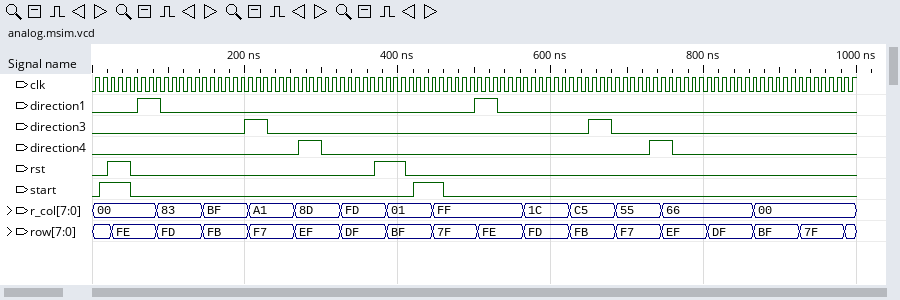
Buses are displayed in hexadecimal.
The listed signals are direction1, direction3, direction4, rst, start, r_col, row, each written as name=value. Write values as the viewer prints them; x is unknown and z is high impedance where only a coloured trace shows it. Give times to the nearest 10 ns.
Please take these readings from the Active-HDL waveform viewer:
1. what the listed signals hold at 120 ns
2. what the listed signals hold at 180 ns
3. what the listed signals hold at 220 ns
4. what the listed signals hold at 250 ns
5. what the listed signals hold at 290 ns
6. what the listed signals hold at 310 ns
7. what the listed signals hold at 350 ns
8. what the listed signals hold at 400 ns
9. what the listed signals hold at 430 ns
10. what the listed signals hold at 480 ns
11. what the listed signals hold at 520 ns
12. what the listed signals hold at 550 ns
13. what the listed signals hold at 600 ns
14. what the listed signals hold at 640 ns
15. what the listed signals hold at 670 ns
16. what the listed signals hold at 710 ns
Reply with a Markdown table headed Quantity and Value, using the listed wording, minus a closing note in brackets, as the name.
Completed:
| Quantity | Value |
|---|---|
| what the listed signals hold at 120 ns | direction1=0, direction3=0, direction4=0, rst=0, start=0, r_col=83, row=FD |
| what the listed signals hold at 180 ns | direction1=0, direction3=0, direction4=0, rst=0, start=0, r_col=BF, row=FB |
| what the listed signals hold at 220 ns | direction1=0, direction3=1, direction4=0, rst=0, start=0, r_col=A1, row=F7 |
| what the listed signals hold at 250 ns | direction1=0, direction3=0, direction4=0, rst=0, start=0, r_col=A1, row=F7 |
| what the listed signals hold at 290 ns | direction1=0, direction3=0, direction4=1, rst=0, start=0, r_col=8D, row=EF |
| what the listed signals hold at 310 ns | direction1=0, direction3=0, direction4=0, rst=0, start=0, r_col=8D, row=EF |
| what the listed signals hold at 350 ns | direction1=0, direction3=0, direction4=0, rst=0, start=0, r_col=FD, row=DF |
| what the listed signals hold at 400 ns | direction1=0, direction3=0, direction4=0, rst=1, start=0, r_col=01, row=BF |
| what the listed signals hold at 430 ns | direction1=0, direction3=0, direction4=0, rst=0, start=1, r_col=01, row=BF |
| what the listed signals hold at 480 ns | direction1=0, direction3=0, direction4=0, rst=0, start=0, r_col=FF, row=7F |
| what the listed signals hold at 520 ns | direction1=1, direction3=0, direction4=0, rst=0, start=0, r_col=FF, row=FE |
| what the listed signals hold at 550 ns | direction1=0, direction3=0, direction4=0, rst=0, start=0, r_col=FF, row=FE |
| what the listed signals hold at 600 ns | direction1=0, direction3=0, direction4=0, rst=0, start=0, r_col=1C, row=FD |
| what the listed signals hold at 640 ns | direction1=0, direction3=0, direction4=0, rst=0, start=0, r_col=C5, row=FB |
| what the listed signals hold at 670 ns | direction1=0, direction3=1, direction4=0, rst=0, start=0, r_col=C5, row=FB |
| what the listed signals hold at 710 ns | direction1=0, direction3=0, direction4=0, rst=0, start=0, r_col=55, row=F7 |
